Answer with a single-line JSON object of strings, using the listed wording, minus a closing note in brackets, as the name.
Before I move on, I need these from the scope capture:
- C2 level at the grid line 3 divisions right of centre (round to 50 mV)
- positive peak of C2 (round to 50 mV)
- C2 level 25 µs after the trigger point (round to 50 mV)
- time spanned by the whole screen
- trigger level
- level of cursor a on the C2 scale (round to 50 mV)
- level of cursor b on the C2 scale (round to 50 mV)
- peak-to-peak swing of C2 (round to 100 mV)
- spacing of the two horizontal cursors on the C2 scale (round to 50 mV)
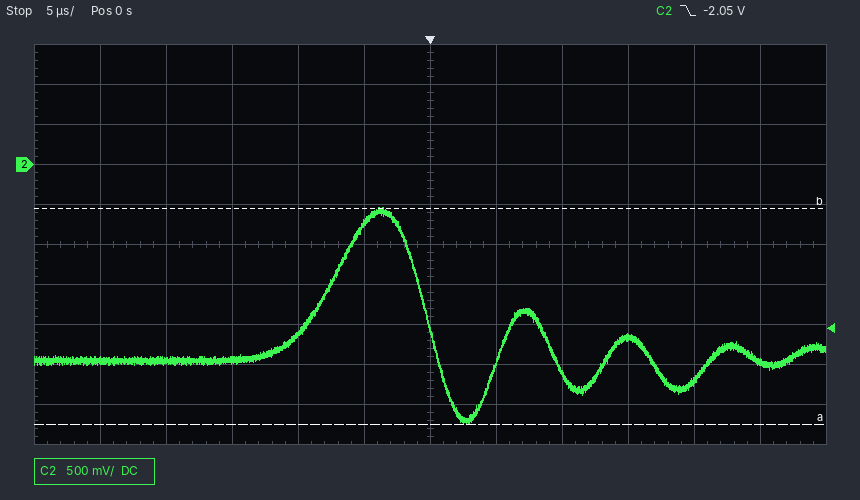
{"C2 level at the grid line 3 divisions right of centre": "-2.15 V", "positive peak of C2": "-550 mV", "C2 level 25 µs after the trigger point": "-2.45 V", "time spanned by the whole screen": "60 µs", "trigger level": "-2.05 V", "level of cursor a on the C2 scale": "-3.25 V", "level of cursor b on the C2 scale": "-550 mV", "peak-to-peak swing of C2": "2.70 V", "spacing of the two horizontal cursors on the C2 scale": "2.70 V"}
